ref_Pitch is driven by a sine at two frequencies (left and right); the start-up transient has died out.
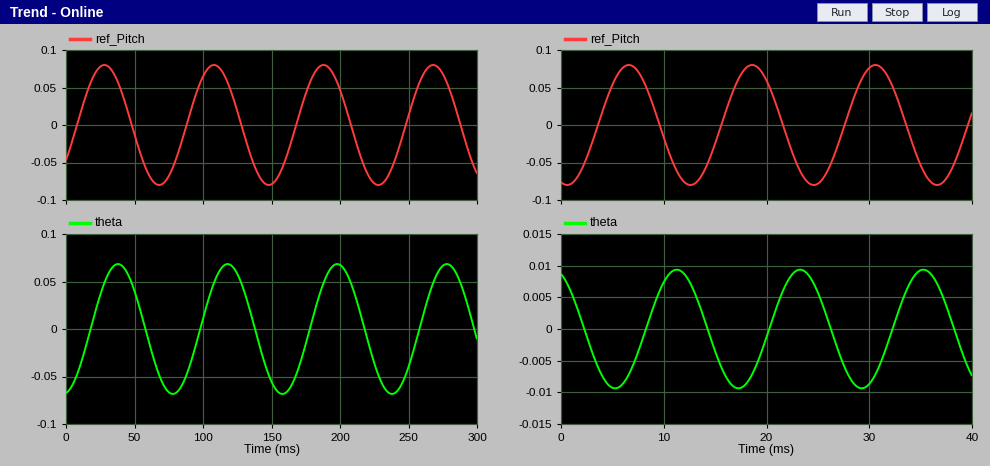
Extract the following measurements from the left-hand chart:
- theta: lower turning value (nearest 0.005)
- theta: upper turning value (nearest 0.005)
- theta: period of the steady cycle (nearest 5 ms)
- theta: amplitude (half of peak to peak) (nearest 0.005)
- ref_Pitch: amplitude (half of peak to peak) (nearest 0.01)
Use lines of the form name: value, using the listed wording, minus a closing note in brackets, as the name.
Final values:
theta: lower turning value: -0.070
theta: upper turning value: 0.070
theta: period of the steady cycle: 80 ms
theta: amplitude (half of peak to peak): 0.070
ref_Pitch: amplitude (half of peak to peak): 0.08
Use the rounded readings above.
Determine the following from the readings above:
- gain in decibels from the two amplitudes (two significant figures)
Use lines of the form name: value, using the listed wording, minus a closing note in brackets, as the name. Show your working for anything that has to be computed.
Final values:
gain in decibels from the two amplitudes: 20 log10(0.07 / 0.08) = -1.2 dB
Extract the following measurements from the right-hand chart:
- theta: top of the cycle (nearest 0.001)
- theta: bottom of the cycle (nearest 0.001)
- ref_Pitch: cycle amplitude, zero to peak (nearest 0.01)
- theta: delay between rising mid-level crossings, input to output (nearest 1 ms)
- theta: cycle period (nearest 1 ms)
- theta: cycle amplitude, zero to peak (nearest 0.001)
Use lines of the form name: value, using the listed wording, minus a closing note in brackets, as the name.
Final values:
theta: top of the cycle: 0.009
theta: bottom of the cycle: -0.009
ref_Pitch: cycle amplitude, zero to peak: 0.08
theta: delay between rising mid-level crossings, input to output: 5 ms
theta: cycle period: 12 ms
theta: cycle amplitude, zero to peak: 0.009
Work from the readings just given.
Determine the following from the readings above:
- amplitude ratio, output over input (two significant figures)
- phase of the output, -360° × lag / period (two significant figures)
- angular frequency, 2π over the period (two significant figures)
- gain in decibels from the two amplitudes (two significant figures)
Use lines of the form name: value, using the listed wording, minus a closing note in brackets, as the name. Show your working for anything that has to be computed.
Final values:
amplitude ratio, output over input: 0.009 / 0.08 = 0.11
phase of the output, -360° × lag / period: -360 × 5 / 12 = -150°
angular frequency, 2π over the period: 2π / 12 = 0.52 rad/ms
gain in decibels from the two amplitudes: 20 log10(0.009 / 0.08) = -19 dB
